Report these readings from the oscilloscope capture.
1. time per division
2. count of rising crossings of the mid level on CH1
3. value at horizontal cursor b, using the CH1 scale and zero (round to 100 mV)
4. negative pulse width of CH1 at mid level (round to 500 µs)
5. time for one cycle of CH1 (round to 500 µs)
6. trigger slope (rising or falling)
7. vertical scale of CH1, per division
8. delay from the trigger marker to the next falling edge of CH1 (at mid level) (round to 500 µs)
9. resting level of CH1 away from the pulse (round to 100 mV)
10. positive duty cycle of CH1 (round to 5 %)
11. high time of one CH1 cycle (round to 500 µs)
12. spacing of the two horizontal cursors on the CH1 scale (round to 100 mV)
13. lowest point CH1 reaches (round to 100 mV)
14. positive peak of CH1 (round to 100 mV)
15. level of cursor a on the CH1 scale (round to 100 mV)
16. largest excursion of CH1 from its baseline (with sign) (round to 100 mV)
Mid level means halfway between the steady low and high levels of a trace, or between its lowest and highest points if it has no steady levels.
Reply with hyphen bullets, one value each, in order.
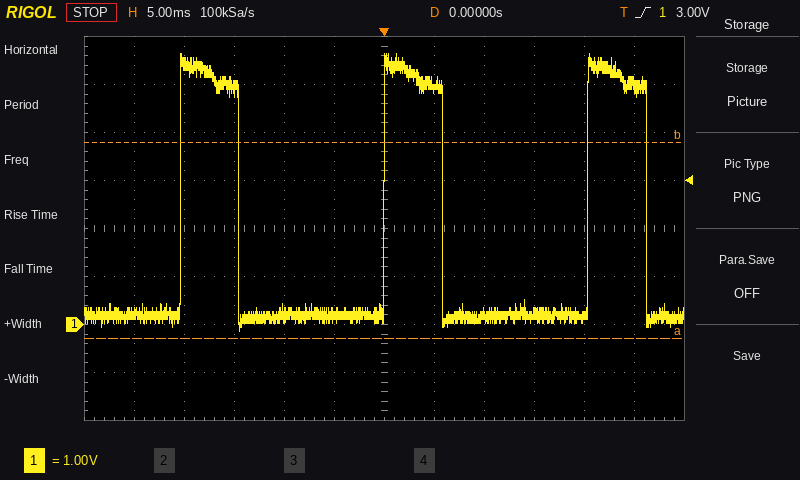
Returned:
- 5 ms
- 3
- 3.8 V
- 14.5 ms
- 20.5 ms
- rising
- 1 V
- 6.0 ms
- 200 mV
- 30 %
- 6.0 ms
- 4.1 V
- -100 mV
- 5.6 V
- -300 mV
- +5.4 V
